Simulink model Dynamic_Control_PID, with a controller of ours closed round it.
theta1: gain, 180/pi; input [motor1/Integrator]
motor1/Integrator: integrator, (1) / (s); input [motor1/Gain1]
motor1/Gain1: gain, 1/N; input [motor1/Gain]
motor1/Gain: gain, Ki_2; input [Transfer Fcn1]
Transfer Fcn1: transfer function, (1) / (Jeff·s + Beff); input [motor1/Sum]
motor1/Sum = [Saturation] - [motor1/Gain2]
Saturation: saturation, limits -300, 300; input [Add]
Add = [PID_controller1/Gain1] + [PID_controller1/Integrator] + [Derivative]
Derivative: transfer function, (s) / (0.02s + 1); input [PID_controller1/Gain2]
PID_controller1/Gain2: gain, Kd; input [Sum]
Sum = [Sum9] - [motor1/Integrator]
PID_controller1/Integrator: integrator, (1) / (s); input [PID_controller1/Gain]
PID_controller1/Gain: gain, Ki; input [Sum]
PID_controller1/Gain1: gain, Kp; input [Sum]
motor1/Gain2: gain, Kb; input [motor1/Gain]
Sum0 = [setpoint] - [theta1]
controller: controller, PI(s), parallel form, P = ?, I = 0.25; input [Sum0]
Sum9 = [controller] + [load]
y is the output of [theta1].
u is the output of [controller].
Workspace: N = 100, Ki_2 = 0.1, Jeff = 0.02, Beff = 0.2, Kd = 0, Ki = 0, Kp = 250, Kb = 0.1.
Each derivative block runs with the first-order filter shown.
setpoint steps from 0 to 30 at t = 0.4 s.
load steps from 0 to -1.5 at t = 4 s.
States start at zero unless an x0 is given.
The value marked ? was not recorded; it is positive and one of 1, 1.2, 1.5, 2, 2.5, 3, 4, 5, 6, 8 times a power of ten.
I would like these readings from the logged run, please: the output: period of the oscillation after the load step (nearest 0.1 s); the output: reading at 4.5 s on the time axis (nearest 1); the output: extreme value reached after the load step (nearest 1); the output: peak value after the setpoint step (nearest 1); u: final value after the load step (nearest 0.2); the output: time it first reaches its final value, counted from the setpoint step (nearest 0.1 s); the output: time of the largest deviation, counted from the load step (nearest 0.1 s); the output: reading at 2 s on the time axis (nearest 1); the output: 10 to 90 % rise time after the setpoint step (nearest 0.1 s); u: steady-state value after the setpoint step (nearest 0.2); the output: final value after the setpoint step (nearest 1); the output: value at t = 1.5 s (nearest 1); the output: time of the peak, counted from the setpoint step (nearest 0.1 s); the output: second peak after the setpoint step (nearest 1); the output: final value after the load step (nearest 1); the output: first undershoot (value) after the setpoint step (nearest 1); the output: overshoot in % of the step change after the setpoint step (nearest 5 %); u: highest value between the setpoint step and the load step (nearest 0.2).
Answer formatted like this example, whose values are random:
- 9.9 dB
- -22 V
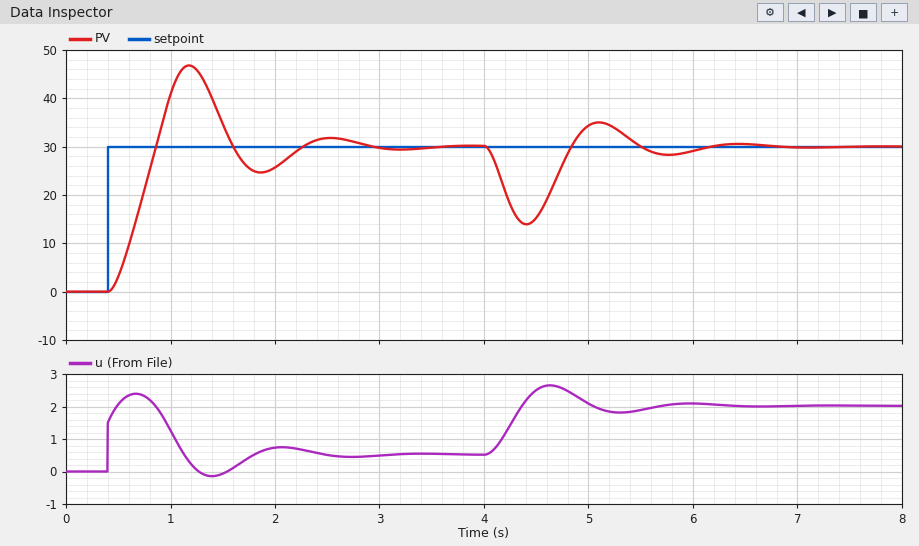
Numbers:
- 1.4 s
- 15
- 14
- 47
- 2.0
- 0.5 s
- 0.4 s
- 26
- 0.3 s
- 0.6
- 30
- 35
- 0.8 s
- 32
- 30
- 25
- 55 %
- 2.4
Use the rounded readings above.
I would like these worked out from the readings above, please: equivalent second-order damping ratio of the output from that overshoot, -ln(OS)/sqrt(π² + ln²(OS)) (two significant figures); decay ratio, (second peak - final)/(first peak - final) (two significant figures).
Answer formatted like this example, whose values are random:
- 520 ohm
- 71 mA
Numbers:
- 0.19
- 0.12
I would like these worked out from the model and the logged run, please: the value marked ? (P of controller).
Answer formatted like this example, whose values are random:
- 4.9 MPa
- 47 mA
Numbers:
- 0.05
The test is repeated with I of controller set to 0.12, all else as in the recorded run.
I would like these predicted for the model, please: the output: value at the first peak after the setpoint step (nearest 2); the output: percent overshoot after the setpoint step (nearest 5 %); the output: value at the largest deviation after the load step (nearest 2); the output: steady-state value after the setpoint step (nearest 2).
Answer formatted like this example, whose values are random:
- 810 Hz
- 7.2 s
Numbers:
- 36
- 20 %
- 12
- 30
